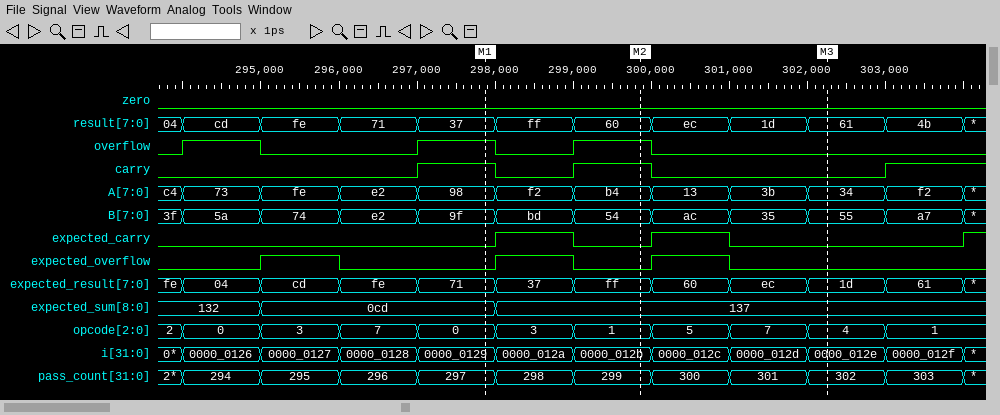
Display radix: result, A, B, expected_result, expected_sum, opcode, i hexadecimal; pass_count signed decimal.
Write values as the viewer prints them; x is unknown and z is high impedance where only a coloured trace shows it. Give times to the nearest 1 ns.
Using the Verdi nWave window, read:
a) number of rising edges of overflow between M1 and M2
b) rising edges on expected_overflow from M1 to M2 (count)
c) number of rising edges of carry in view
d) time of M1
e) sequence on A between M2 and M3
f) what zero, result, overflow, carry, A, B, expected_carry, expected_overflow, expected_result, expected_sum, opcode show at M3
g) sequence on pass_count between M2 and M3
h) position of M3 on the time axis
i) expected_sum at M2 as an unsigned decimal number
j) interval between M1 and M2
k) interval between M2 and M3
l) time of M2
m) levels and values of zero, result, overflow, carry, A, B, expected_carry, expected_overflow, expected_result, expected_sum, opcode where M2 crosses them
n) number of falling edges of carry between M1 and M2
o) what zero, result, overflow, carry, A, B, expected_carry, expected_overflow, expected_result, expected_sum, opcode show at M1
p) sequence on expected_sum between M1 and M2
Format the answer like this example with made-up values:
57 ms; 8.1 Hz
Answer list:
1; 1; 3; 298 ns; b4, 13, 3b, 34; zero=0, result=61, overflow=0, carry=0, A=34, B=55, expected_carry=0, expected_overflow=0, expected_result=1d, expected_sum=137, opcode=4; 299, 300, 301, 302; 302 ns; 311; 2 ns; 2 ns; 300 ns; zero=0, result=60, overflow=1, carry=1, A=b4, B=54, expected_carry=0, expected_overflow=0, expected_result=ff, expected_sum=137, opcode=1; 1; zero=0, result=37, overflow=1, carry=1, A=98, B=9f, expected_carry=0, expected_overflow=0, expected_result=71, expected_sum=0cd, opcode=0; 0cd, 137
